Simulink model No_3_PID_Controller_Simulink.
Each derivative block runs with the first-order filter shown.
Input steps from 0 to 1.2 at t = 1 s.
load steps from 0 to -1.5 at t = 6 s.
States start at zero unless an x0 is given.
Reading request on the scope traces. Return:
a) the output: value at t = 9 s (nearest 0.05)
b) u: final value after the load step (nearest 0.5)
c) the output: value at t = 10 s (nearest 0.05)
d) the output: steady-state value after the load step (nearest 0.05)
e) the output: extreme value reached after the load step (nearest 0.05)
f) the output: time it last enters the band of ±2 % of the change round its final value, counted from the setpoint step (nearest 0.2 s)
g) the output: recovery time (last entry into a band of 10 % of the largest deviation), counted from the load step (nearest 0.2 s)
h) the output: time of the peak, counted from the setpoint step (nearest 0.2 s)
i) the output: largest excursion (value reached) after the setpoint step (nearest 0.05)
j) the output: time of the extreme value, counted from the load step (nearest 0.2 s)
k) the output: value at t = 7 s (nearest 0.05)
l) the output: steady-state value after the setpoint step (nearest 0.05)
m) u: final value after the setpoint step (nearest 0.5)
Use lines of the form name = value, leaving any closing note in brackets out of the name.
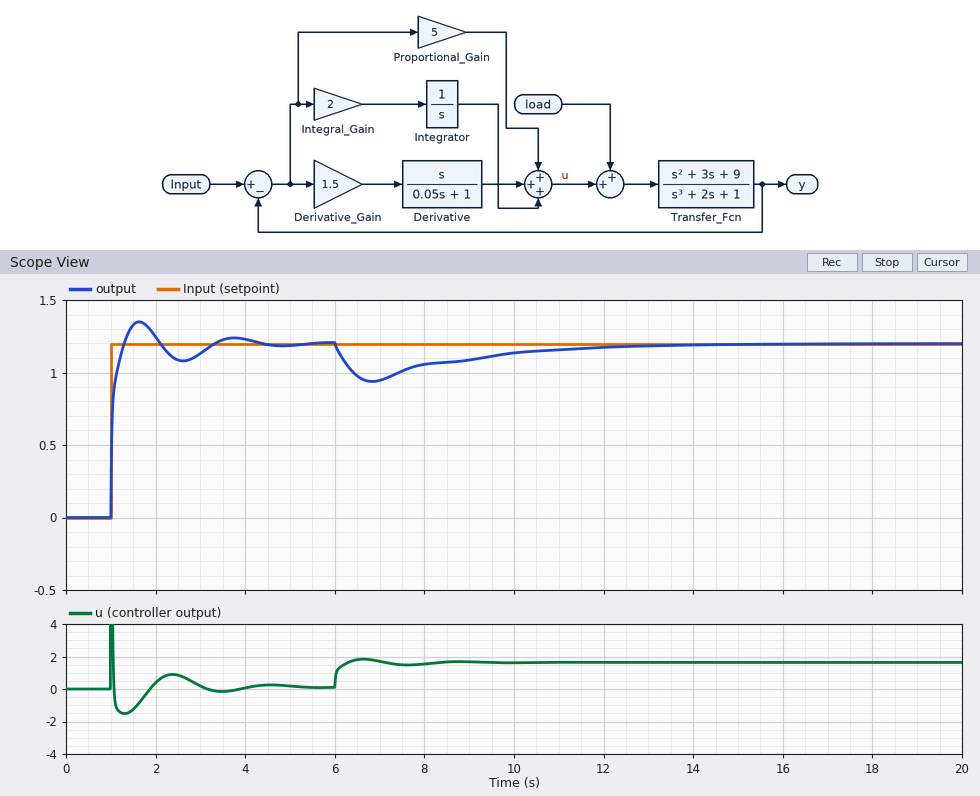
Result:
the output: value at t = 9 s = 1.10
u: final value after the load step = 1.5
the output: value at t = 10 s = 1.15
the output: steady-state value after the load step = 1.20
the output: extreme value reached after the load step = 0.95
the output: time it last enters the band of ±2 % of the change round its final value, counted from the setpoint step = 3.0 s
the output: recovery time (last entry into a band of 10 % of the largest deviation), counted from the load step = 6.0 s
the output: time of the peak, counted from the setpoint step = 0.6 s
the output: largest excursion (value reached) after the setpoint step = 1.35
the output: time of the extreme value, counted from the load step = 0.8 s
the output: value at t = 7 s = 0.95
the output: steady-state value after the setpoint step = 1.20
u: final value after the setpoint step = 0.0
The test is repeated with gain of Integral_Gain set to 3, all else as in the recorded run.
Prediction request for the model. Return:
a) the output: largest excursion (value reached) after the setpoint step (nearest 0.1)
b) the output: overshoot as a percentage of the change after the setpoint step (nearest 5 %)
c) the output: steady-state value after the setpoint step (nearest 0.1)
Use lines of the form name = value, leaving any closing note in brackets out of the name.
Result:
the output: largest excursion (value reached) after the setpoint step = 1.4
the output: overshoot as a percentage of the change after the setpoint step = 15 %
the output: steady-state value after the setpoint step = 1.2
